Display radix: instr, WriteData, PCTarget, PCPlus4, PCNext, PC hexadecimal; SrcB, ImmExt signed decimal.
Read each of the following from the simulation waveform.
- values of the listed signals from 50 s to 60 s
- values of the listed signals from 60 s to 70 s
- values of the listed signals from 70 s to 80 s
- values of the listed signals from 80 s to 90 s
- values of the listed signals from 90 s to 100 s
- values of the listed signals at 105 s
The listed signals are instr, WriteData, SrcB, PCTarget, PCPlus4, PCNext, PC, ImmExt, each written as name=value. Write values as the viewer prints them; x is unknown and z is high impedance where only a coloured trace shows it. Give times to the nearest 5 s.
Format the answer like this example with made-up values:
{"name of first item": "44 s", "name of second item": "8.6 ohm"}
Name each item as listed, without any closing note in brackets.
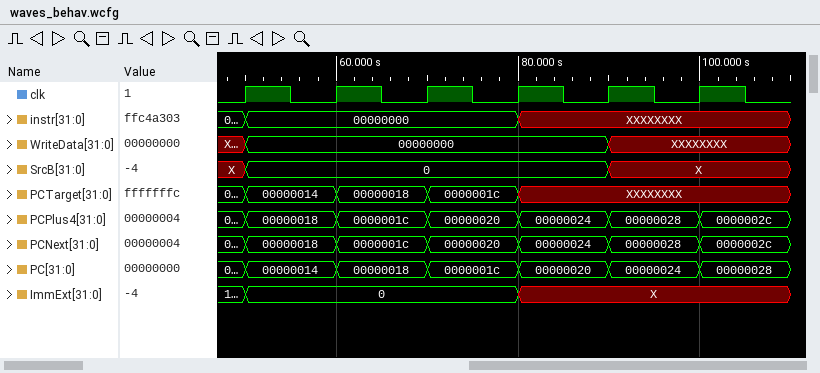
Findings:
{"values of the listed signals from 50 s to 60 s": "instr=00000000, WriteData=00000000, SrcB=0, PCTarget=00000014, PCPlus4=00000018, PCNext=00000018, PC=00000014, ImmExt=0", "values of the listed signals from 60 s to 70 s": "instr=00000000, WriteData=00000000, SrcB=0, PCTarget=00000018, PCPlus4=0000001c, PCNext=0000001c, PC=00000018, ImmExt=0", "values of the listed signals from 70 s to 80 s": "instr=00000000, WriteData=00000000, SrcB=0, PCTarget=0000001c, PCPlus4=00000020, PCNext=00000020, PC=0000001c, ImmExt=0", "values of the listed signals from 80 s to 90 s": "instr=XXXXXXXX, WriteData=00000000, SrcB=0, PCTarget=XXXXXXXX, PCPlus4=00000024, PCNext=00000024, PC=00000020, ImmExt=X", "values of the listed signals from 90 s to 100 s": "instr=XXXXXXXX, WriteData=XXXXXXXX, SrcB=X, PCTarget=XXXXXXXX, PCPlus4=00000028, PCNext=00000028, PC=00000024, ImmExt=X", "values of the listed signals at 105 s": "instr=XXXXXXXX, WriteData=XXXXXXXX, SrcB=X, PCTarget=XXXXXXXX, PCPlus4=0000002c, PCNext=0000002c, PC=00000028, ImmExt=X"}
